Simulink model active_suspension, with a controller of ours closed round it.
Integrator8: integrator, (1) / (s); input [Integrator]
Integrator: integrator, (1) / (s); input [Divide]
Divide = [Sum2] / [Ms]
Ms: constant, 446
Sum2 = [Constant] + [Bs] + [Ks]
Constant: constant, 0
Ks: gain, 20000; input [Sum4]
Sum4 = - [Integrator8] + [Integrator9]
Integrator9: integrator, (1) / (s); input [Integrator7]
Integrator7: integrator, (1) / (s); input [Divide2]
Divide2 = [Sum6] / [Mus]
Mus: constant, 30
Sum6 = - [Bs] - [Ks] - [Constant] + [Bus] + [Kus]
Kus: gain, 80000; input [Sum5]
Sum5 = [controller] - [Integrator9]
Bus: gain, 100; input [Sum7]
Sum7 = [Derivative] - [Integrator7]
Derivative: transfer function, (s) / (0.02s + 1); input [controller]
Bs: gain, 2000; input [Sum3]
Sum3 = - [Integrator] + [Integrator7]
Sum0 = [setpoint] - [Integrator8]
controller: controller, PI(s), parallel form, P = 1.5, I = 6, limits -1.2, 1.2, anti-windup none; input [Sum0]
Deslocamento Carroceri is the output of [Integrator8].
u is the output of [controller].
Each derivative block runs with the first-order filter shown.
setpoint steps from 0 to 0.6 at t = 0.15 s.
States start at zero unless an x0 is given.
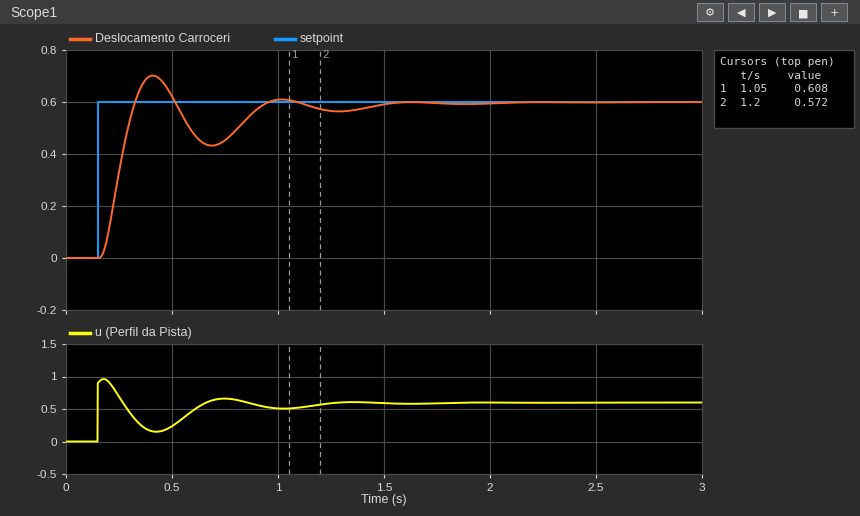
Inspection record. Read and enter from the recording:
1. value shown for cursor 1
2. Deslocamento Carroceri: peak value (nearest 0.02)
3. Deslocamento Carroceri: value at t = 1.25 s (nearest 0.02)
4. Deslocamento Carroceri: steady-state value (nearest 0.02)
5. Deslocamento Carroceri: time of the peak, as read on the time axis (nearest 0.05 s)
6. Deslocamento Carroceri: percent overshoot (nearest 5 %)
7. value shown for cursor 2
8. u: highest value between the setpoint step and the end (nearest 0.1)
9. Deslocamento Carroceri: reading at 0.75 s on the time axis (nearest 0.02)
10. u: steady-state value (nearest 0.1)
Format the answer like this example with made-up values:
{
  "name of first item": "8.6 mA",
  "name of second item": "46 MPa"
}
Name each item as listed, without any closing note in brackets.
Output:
{
  "value shown for cursor 1": "0.608",
  "Deslocamento Carroceri: peak value": "0.70",
  "Deslocamento Carroceri: value at t = 1.25 s": "0.56",
  "Deslocamento Carroceri: steady-state value": "0.60",
  "Deslocamento Carroceri: time of the peak, as read on the time axis": "0.40 s",
  "Deslocamento Carroceri: percent overshoot": "15 %",
  "value shown for cursor 2": "0.572",
  "u: highest value between the setpoint step and the end": "1.0",
  "Deslocamento Carroceri: reading at 0.75 s on the time axis": "0.46",
  "u: steady-state value": "0.6"
}
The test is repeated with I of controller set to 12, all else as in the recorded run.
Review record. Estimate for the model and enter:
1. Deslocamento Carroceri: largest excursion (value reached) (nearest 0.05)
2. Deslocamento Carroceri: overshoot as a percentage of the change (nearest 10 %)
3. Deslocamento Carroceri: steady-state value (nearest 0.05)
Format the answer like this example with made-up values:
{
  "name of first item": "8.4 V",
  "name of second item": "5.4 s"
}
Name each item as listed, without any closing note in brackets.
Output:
{
  "Deslocamento Carroceri: largest excursion (value reached)": "0.85",
  "Deslocamento Carroceri: overshoot as a percentage of the change": "40 %",
  "Deslocamento Carroceri: steady-state value": "0.60"
}
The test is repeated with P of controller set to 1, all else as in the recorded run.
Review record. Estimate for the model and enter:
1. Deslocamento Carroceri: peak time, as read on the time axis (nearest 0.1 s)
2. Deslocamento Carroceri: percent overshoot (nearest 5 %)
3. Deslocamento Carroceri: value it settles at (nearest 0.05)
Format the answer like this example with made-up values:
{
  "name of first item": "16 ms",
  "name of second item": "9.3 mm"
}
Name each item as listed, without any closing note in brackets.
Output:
{
  "Deslocamento Carroceri: peak time, as read on the time axis": "0.5 s",
  "Deslocamento Carroceri: percent overshoot": "20 %",
  "Deslocamento Carroceri: value it settles at": "0.60"
}
